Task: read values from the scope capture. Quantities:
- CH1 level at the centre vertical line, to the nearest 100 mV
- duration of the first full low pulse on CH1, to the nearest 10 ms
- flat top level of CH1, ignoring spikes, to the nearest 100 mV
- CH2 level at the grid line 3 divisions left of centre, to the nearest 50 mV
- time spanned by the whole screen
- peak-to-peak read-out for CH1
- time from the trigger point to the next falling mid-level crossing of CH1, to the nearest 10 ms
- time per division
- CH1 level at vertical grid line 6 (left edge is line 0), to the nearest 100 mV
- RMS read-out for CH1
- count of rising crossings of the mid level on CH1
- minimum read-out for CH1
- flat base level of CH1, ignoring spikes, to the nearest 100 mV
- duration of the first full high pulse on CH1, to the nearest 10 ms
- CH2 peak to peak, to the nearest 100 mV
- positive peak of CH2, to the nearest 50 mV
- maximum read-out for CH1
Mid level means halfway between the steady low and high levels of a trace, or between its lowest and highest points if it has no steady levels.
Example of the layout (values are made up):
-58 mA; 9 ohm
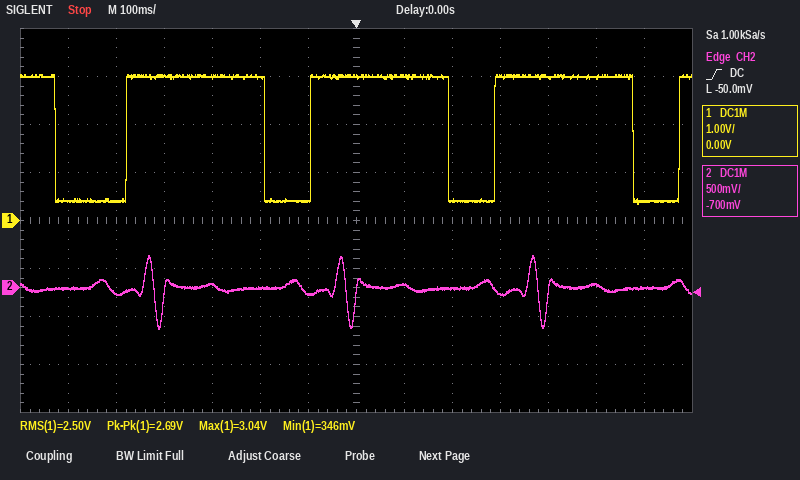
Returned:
3.0 V; 150 ms; 3.0 V; 50 mV; 1.4 s; 2.69 V; 190 ms; 100 ms; 400 mV; 2.50 V; 4; 346 mV; 400 mV; 290 ms; 800 mV; 350 mV; 3.04 V
